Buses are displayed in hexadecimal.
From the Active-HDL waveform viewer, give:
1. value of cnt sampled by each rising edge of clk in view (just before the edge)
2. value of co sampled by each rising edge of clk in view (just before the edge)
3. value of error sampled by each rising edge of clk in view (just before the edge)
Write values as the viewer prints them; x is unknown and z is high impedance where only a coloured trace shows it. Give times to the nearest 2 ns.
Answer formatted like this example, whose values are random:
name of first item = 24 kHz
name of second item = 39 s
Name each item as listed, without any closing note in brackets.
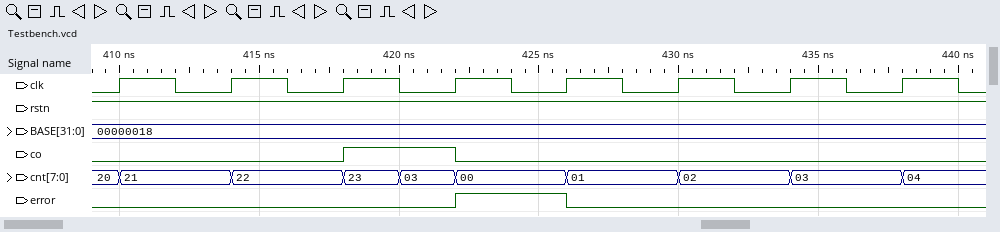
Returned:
value of cnt sampled by each rising edge of clk in view = 20, 21, 22, 03, 00, 01, 02, 03
value of co sampled by each rising edge of clk in view = 0 0 0 1 0 0 0 0
value of error sampled by each rising edge of clk in view = 0 0 0 0 1 0 0 0
